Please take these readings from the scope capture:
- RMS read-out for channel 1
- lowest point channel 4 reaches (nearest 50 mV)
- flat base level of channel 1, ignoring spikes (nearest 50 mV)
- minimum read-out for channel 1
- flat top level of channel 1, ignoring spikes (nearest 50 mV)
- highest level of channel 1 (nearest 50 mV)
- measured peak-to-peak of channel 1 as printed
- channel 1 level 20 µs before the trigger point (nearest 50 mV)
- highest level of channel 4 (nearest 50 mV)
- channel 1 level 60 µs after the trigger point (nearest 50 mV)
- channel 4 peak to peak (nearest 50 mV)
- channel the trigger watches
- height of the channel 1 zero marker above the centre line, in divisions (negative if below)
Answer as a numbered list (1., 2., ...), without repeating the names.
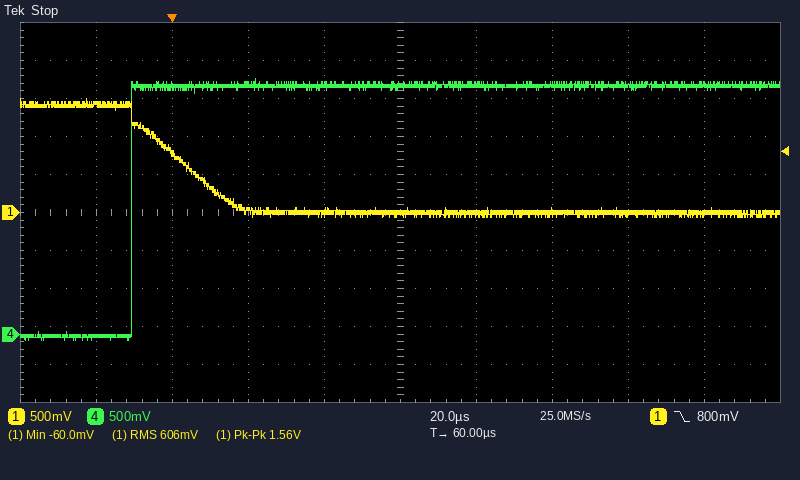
1. 606 mV
2. -100 mV
3. 0 mV
4. -60.0 mV
5. 1.40 V
6. 1.50 V
7. 1.56 V
8. 1.40 V
9. 3.35 V
10. 0 mV
11. 3.45 V
12. channel 1
13. 0.0 div
